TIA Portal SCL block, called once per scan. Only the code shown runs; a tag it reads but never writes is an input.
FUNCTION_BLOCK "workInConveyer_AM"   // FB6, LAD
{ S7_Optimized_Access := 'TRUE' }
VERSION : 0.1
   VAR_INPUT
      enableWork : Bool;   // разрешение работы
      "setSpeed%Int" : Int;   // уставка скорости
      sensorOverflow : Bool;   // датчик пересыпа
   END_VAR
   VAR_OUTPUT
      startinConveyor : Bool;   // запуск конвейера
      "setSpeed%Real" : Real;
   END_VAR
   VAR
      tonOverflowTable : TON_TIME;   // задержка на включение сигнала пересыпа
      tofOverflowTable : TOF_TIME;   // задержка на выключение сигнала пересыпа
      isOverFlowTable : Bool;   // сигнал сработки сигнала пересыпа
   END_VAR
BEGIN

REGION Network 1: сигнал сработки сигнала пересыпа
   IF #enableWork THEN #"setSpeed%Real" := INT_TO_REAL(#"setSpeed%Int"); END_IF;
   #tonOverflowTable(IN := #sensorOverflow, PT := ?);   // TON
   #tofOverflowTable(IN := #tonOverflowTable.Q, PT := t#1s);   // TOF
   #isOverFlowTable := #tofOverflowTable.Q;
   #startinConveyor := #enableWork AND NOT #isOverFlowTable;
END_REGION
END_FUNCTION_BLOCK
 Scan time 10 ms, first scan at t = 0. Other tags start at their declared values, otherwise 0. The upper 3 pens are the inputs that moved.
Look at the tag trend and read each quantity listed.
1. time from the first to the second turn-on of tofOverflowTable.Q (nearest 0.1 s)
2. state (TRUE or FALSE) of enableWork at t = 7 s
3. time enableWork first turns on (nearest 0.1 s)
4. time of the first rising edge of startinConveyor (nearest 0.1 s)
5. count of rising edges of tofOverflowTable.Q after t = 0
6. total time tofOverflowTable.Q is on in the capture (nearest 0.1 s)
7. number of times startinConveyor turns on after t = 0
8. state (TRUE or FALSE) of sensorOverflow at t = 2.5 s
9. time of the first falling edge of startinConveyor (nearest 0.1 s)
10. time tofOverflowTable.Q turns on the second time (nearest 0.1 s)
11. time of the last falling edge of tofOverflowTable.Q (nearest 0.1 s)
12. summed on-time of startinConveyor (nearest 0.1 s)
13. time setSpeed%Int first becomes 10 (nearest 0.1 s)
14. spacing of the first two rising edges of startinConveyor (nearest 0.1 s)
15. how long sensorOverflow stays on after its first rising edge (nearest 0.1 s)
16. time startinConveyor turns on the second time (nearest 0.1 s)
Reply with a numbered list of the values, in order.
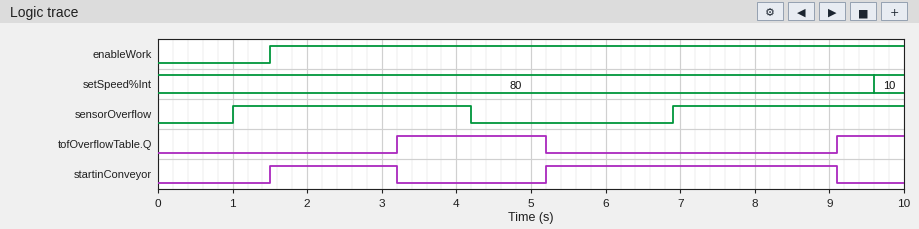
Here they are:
1. 5.9 s
2. TRUE
3. 1.5 s
4. 1.5 s
5. 2
6. 2.9 s
7. 2
8. TRUE
9. 3.2 s
10. 9.1 s
11. 5.2 s
12. 5.6 s
13. 9.6 s
14. 3.7 s
15. 3.2 s
16. 5.2 s
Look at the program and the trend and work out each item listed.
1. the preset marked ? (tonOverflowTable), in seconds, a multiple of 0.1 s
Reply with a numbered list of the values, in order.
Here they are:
1. 2.2 s
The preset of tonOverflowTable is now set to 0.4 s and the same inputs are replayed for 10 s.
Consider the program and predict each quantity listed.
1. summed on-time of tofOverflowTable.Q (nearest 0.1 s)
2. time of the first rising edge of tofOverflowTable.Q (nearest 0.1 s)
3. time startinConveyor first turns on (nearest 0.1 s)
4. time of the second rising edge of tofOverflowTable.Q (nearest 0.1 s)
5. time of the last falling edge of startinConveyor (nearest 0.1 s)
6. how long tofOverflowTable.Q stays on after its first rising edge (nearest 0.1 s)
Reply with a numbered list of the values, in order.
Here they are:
1. 6.5 s
2. 1.4 s
3. 5.2 s
4. 7.3 s
5. 7.3 s
6. 3.8 s
